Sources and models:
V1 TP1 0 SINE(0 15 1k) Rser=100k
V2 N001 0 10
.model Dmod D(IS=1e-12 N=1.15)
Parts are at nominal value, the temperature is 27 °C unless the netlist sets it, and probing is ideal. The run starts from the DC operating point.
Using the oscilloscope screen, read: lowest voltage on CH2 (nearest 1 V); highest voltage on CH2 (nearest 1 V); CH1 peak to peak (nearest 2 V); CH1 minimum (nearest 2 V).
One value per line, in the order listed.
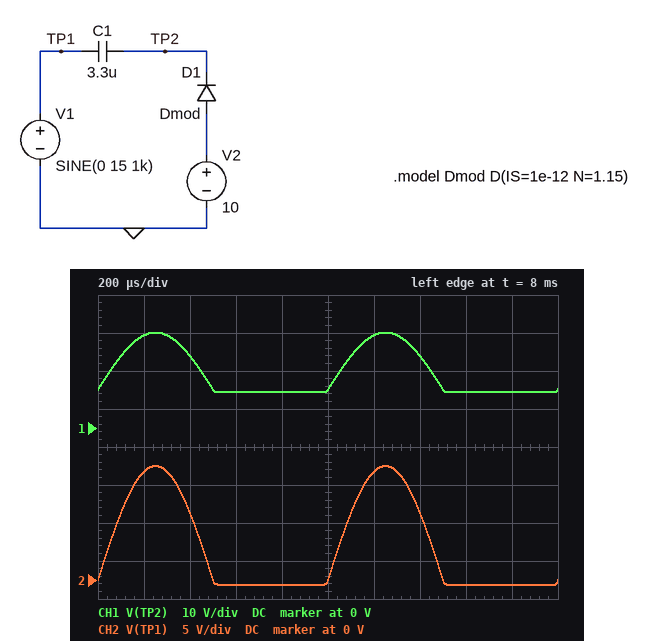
-1 V
15 V
16 V
10 V
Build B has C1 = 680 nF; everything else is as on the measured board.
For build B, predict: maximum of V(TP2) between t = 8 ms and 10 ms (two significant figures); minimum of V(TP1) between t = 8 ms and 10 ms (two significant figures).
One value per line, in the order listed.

26 V
-1.2 V
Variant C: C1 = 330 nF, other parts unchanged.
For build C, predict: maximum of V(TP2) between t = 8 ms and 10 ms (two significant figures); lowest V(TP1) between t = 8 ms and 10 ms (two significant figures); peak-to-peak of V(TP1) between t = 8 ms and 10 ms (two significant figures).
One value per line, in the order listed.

26 V
-1.8 V
17 V
